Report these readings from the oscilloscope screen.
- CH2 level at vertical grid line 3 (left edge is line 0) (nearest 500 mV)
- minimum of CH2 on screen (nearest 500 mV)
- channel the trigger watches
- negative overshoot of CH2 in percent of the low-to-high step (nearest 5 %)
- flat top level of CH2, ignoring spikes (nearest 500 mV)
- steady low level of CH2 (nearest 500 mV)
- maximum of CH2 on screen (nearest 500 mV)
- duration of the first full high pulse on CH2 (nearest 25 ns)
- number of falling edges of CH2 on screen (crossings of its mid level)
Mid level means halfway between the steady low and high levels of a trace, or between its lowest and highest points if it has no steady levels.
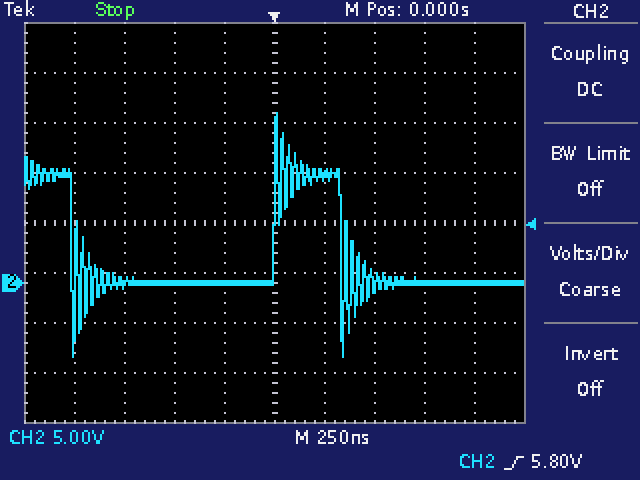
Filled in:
0.0 V
-7.5 V
CH2
65 %
11.0 V
0.0 V
17.0 V
325 ns
2
